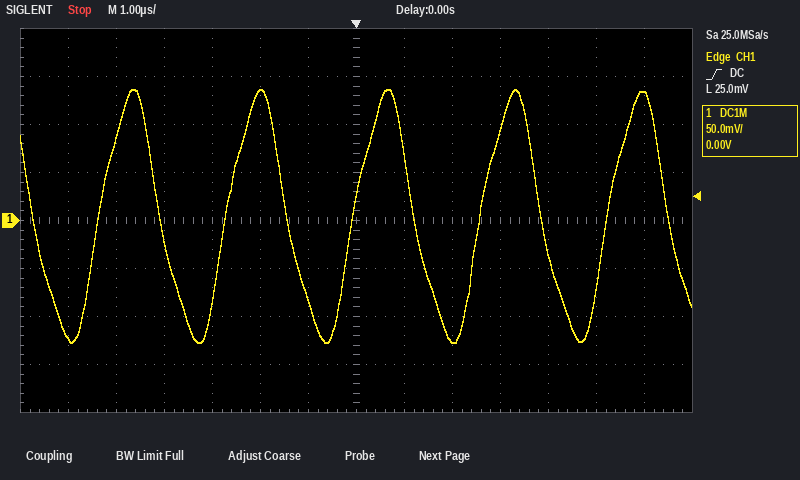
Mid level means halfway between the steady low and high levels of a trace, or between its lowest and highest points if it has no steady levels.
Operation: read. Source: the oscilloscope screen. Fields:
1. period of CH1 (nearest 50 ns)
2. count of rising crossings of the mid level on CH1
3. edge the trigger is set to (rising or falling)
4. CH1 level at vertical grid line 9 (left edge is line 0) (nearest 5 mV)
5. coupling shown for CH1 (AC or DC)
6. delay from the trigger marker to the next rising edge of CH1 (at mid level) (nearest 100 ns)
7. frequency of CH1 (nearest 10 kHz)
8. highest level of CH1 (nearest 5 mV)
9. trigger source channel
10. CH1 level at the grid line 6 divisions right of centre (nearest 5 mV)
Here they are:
2.65 µs
5
rising
-125 mV
DC
2.6 µs
380 kHz
135 mV
CH1
135 mV
